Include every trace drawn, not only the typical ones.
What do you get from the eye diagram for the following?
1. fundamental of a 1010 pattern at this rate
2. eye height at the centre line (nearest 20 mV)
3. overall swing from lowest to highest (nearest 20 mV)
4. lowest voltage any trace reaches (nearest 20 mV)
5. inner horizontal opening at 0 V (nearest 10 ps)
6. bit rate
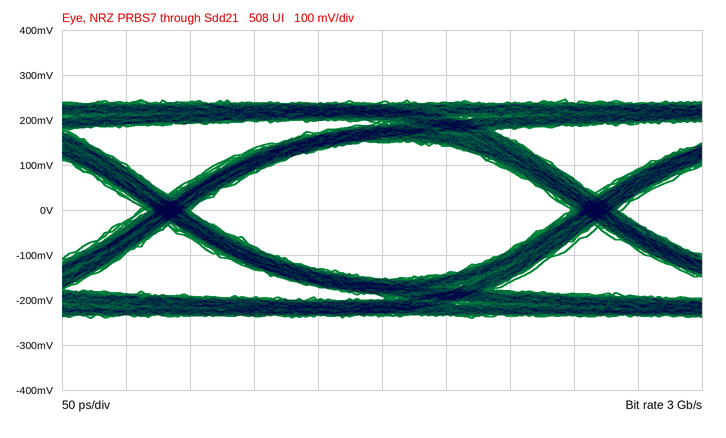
1.5 GHz
300 mV
480 mV
-240 mV
300 ps
3 Gb/s
